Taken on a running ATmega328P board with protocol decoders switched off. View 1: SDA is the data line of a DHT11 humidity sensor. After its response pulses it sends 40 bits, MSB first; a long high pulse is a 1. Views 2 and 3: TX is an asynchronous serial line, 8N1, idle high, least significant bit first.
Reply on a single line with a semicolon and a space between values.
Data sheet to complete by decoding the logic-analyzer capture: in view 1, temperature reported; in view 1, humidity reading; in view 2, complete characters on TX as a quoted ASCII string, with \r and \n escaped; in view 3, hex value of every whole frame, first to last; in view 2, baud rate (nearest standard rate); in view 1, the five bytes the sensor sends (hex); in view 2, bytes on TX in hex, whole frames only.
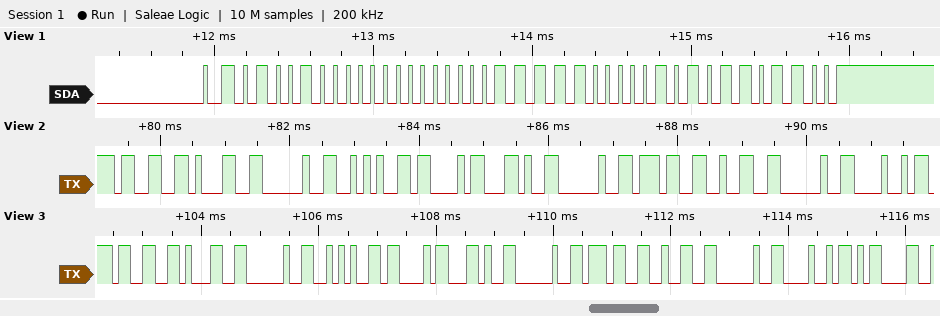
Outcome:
31.5 °C; 72 %; "31 *C, 72 H"; 0x33 0x31 0x20 0x2A 0x43 0x2C 0x20 0x37 0x32 0x20 0x48 0x0D; 9600 baud; 48 00 1F 05 6C; 0x33 0x31 0x20 0x2A 0x43 0x2C 0x20 0x37 0x32 0x20 0x48
